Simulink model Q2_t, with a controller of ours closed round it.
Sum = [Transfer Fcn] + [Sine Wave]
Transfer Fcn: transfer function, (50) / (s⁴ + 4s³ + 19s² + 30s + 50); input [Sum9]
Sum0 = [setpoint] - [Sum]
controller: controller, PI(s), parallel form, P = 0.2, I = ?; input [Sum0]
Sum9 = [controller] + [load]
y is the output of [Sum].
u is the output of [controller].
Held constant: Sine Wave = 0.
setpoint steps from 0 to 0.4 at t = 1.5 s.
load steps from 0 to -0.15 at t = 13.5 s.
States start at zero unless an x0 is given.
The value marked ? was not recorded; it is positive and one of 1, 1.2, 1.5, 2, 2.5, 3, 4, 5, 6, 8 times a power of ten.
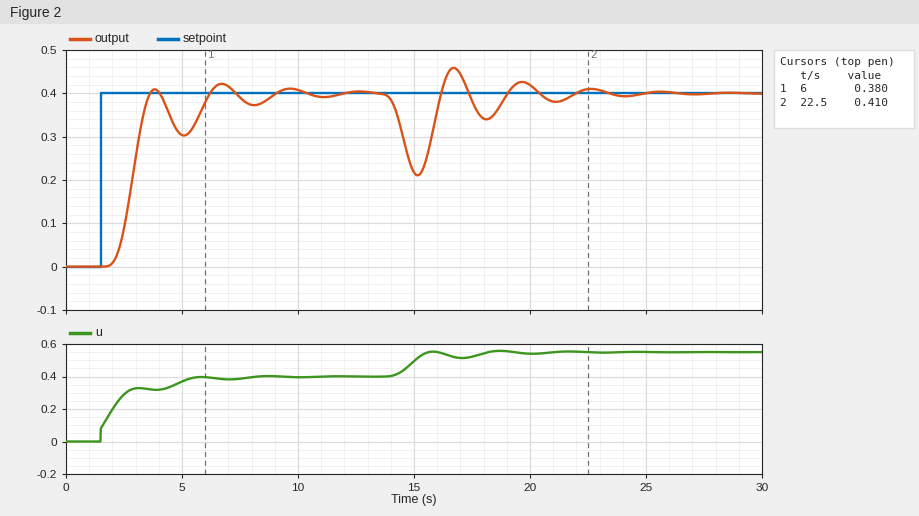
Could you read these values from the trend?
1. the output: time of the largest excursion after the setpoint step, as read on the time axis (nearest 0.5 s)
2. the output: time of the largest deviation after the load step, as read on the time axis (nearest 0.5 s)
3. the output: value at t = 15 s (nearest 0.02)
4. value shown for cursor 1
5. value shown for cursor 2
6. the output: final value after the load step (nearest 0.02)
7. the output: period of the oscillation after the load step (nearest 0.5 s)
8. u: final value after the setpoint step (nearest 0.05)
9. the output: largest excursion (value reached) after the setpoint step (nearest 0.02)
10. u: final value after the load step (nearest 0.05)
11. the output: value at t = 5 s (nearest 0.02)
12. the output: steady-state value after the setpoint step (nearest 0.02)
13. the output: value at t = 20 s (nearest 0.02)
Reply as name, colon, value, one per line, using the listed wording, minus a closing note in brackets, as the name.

the output: time of the largest excursion after the setpoint step, as read on the time axis: 6.5 s
the output: time of the largest deviation after the load step, as read on the time axis: 15.0 s
the output: value at t = 15 s: 0.22
value shown for cursor 1: 0.380
value shown for cursor 2: 0.410
the output: final value after the load step: 0.40
the output: period of the oscillation after the load step: 3.0 s
u: final value after the setpoint step: 0.40
the output: largest excursion (value reached) after the setpoint step: 0.42
u: final value after the load step: 0.55
the output: value at t = 5 s: 0.30
the output: steady-state value after the setpoint step: 0.40
the output: value at t = 20 s: 0.42
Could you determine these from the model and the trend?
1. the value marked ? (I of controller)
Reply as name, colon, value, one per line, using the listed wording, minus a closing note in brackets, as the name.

the value marked ?: 0.6
